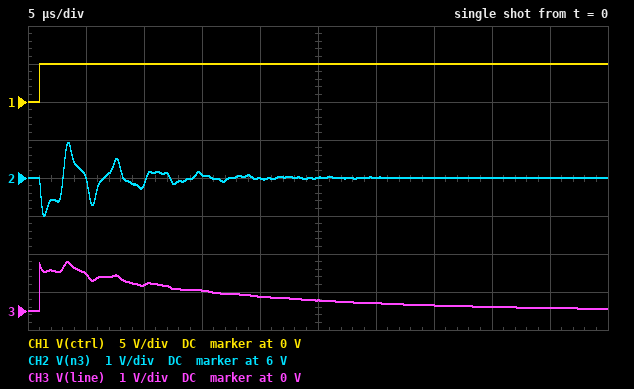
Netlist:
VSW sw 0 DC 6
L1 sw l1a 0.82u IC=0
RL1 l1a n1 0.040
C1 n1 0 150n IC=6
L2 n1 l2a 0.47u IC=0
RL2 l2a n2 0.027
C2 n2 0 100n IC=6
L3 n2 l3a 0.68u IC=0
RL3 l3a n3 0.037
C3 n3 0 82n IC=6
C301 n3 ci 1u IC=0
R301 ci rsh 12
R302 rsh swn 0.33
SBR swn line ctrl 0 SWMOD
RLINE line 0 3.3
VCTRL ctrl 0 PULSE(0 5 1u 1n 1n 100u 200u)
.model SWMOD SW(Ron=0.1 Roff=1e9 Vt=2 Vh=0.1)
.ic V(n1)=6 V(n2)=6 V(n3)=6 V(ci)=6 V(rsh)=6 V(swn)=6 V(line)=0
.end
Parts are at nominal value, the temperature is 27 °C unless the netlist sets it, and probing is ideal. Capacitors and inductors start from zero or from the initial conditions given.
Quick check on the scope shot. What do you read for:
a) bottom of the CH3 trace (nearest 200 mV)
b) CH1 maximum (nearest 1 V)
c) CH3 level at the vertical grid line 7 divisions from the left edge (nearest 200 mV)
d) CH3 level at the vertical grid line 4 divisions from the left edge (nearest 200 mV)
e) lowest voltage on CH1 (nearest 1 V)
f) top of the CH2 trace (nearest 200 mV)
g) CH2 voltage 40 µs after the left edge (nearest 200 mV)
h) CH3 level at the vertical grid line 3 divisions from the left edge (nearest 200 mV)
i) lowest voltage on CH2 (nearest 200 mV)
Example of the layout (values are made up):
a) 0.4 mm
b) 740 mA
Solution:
a) 0 V
b) 5 V
c) 200 mV
d) 400 mV
e) 0 V
f) 7.0 V
g) 6.0 V
h) 600 mV
i) 5.0 V
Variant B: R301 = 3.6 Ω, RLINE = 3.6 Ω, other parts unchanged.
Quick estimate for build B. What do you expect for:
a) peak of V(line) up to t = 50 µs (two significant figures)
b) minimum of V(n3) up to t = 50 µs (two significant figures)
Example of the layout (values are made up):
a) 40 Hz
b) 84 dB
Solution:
a) 2.8 V
b) 4.2 V
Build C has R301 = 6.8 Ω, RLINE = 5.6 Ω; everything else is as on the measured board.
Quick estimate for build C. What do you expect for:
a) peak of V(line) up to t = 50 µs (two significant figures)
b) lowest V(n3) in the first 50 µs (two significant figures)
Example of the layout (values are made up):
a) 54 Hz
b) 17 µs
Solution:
a) 2.7 V
b) 4.8 V
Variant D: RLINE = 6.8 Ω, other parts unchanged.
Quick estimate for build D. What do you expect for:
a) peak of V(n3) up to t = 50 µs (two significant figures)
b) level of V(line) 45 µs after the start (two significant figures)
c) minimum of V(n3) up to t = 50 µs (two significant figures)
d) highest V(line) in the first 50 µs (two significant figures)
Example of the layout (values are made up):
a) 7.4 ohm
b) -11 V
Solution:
a) 6.8 V
b) 220 mV
c) 5.2 V
d) 2.2 V
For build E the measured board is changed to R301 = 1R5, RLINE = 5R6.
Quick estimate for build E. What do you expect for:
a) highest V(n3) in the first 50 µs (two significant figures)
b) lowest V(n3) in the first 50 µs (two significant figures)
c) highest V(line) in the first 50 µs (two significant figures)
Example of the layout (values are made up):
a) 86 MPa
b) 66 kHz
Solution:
a) 7.4 V
b) 4.2 V
c) 4.5 V
